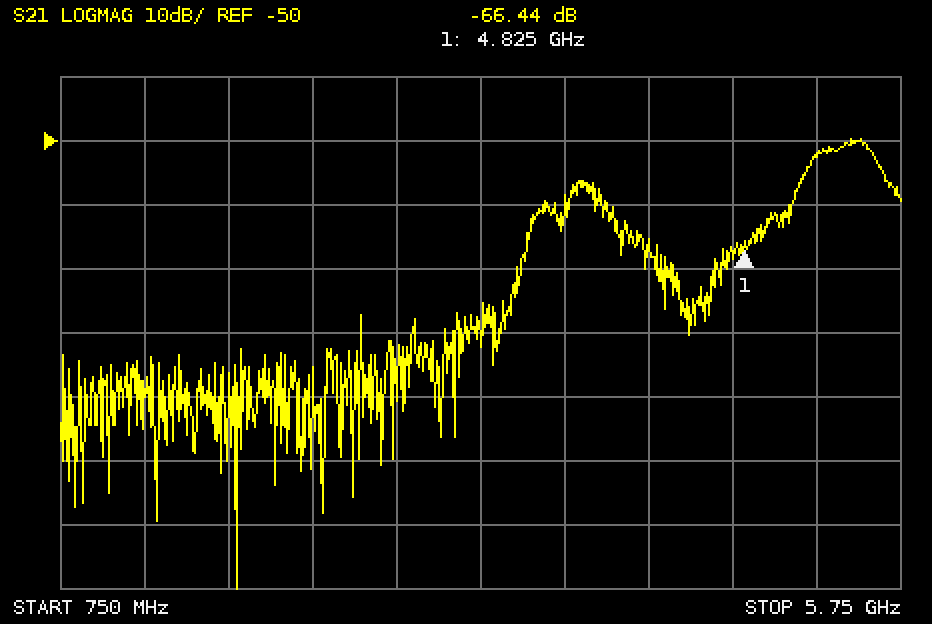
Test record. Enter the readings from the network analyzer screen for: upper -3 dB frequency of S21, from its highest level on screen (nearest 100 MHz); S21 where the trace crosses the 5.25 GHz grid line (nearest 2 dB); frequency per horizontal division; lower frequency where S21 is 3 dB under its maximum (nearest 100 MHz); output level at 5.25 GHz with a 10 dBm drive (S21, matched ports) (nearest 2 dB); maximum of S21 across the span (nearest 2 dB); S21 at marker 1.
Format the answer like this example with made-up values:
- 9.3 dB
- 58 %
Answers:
- 5.6 GHz
- -52 dB
- 500 MHz
- 5.2 GHz
- -42 dBm
- -50 dB
- -66.44 dB
